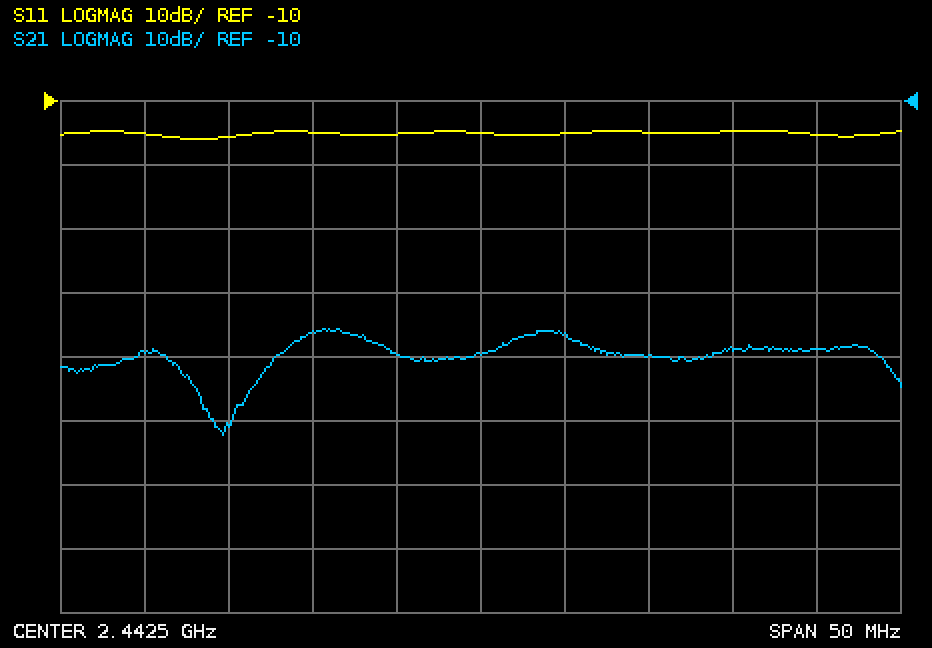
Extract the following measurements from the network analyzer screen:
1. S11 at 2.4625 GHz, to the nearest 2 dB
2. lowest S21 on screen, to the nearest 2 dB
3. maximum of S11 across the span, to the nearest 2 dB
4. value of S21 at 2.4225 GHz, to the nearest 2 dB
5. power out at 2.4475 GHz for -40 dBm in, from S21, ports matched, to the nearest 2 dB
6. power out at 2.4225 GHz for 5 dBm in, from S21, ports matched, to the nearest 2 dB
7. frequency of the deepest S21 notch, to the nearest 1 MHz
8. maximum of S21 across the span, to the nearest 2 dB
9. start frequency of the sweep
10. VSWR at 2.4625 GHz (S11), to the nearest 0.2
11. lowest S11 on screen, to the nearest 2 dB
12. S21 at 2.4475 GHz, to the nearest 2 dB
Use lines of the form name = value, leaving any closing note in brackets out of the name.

S11 at 2.4625 GHz, to the nearest 2 dB = -16 dB
lowest S21 on screen, to the nearest 2 dB = -62 dB
maximum of S11 across the span, to the nearest 2 dB = -14 dB
value of S21 at 2.4225 GHz, to the nearest 2 dB = -50 dB
power out at 2.4475 GHz for -40 dBm in, from S21, ports matched, to the nearest 2 dB = -86 dBm
power out at 2.4225 GHz for 5 dBm in, from S21, ports matched, to the nearest 2 dB = -44 dBm
frequency of the deepest S21 notch, to the nearest 1 MHz = 2.427 GHz
maximum of S21 across the span, to the nearest 2 dB = -46 dB
start frequency of the sweep = 2.4175 GHz
VSWR at 2.4625 GHz (S11), to the nearest 0.2 = 1.4
lowest S11 on screen, to the nearest 2 dB = -16 dB
S21 at 2.4475 GHz, to the nearest 2 dB = -46 dB
